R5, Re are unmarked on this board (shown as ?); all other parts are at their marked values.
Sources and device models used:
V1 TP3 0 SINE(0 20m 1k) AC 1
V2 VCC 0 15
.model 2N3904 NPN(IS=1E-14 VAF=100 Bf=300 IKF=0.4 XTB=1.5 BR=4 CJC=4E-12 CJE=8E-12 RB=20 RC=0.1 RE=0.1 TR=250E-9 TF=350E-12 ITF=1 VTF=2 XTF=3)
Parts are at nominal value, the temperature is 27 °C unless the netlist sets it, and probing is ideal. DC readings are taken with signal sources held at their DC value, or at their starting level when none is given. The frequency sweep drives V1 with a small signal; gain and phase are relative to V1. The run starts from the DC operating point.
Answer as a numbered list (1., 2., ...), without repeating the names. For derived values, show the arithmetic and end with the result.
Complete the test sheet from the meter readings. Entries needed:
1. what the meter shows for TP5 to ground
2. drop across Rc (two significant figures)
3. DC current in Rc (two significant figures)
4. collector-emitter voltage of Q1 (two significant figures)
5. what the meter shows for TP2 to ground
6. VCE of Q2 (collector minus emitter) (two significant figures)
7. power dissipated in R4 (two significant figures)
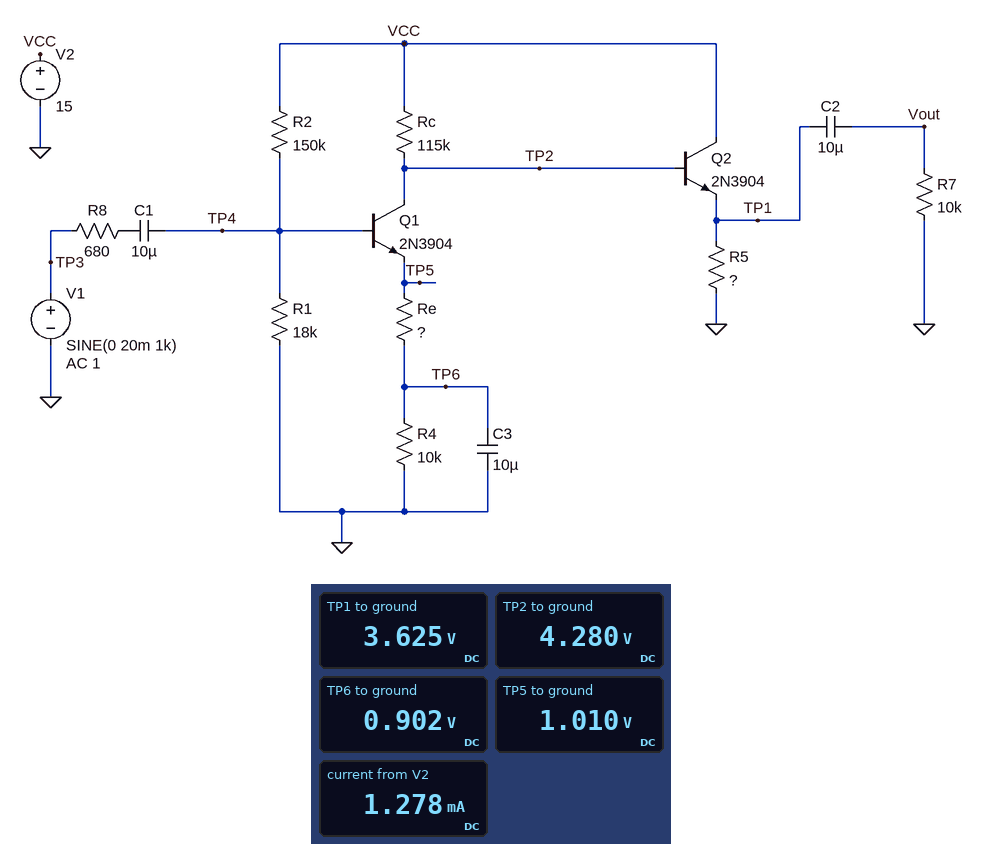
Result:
1. 1.010 V
2. 15 V - 4.28 V = 11 V
3. (15 V - 4.28 V) / 115 kΩ = 93 µA
4. 4.28 V - 1.01 V = 3.3 V
5. 4.280 V
6. 15 V - 3.625 V = 11 V
7. (902 mV)^2 / 10 kΩ = 81 µW
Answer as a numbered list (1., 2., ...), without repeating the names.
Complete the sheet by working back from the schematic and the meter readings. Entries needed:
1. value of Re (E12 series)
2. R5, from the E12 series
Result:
1. 1.2 kΩ
2. 3.3 kΩ
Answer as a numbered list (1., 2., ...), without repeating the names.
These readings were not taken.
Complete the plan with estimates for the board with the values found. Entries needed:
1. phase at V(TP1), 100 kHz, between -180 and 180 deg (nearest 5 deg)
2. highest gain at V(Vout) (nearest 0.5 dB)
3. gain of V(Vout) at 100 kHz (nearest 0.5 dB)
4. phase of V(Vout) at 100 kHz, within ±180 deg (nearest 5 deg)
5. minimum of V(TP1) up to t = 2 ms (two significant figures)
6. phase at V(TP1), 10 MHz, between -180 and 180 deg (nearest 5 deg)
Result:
1. 160 deg
2. 36.0 dB
3. 35.5 dB
4. 160 deg
5. 2.4 V
6. 65 deg
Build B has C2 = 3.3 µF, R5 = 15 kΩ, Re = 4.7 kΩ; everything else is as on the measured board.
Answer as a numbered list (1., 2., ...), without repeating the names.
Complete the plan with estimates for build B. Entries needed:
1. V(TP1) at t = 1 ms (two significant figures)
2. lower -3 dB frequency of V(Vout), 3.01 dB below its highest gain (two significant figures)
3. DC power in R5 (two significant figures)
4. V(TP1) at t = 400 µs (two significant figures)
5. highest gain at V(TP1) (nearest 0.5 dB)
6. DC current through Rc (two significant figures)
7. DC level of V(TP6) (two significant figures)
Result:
1. 6.3 V
2. 7.1 Hz
3. 2.6 mW
4. 6.0 V
5. 26.0 dB
6. 70 µA
7. 690 mV
